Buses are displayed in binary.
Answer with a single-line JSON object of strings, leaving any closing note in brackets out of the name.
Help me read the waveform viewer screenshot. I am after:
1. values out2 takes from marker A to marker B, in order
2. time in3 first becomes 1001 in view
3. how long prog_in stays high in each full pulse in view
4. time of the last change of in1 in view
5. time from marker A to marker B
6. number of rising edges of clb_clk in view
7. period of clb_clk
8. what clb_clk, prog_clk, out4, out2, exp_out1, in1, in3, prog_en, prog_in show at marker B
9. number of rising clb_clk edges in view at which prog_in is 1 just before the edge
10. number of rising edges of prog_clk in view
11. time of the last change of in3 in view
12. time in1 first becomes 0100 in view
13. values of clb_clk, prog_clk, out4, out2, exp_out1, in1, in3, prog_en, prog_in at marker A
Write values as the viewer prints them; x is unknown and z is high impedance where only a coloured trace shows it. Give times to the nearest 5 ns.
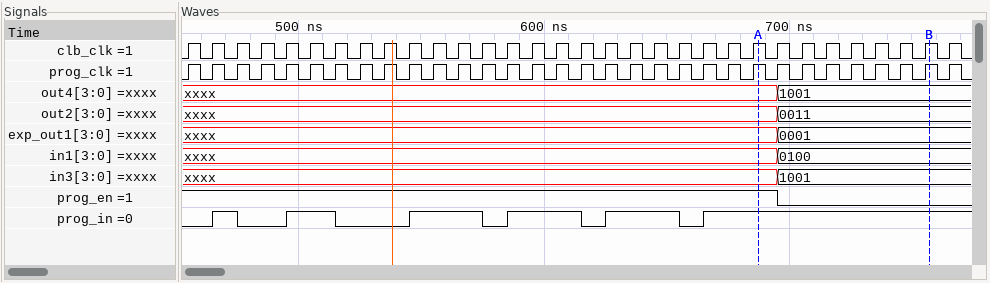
{"values out2 takes from marker A to marker B, in order": "xxxx, 0011", "time in3 first becomes 1001 in view": "695 ns", "how long prog_in stays high in each full pulse in view": "10 ns, 20 ns, 30 ns, 30 ns, 30 ns", "time of the last change of in1 in view": "695 ns", "time from marker A to marker B": "70 ns", "number of rising edges of clb_clk in view": "32", "period of clb_clk": "10 ns", "what clb_clk, prog_clk, out4, out2, exp_out1, in1, in3, prog_en, prog_in show at marker B": "clb_clk=1, prog_clk=1, out4=1001, out2=0011, exp_out1=0001, in1=0100, in3=1001, prog_en=0, prog_in=1", "number of rising clb_clk edges in view at which prog_in is 1 just before the edge": "22", "number of rising edges of prog_clk in view": "32", "time of the last change of in3 in view": "695 ns", "time in1 first becomes 0100 in view": "695 ns", "values of clb_clk, prog_clk, out4, out2, exp_out1, in1, in3, prog_en, prog_in at marker A": "clb_clk=1, prog_clk=1, out4=xxxx, out2=xxxx, exp_out1=xxxx, in1=xxxx, in3=xxxx, prog_en=1, prog_in=1"}
